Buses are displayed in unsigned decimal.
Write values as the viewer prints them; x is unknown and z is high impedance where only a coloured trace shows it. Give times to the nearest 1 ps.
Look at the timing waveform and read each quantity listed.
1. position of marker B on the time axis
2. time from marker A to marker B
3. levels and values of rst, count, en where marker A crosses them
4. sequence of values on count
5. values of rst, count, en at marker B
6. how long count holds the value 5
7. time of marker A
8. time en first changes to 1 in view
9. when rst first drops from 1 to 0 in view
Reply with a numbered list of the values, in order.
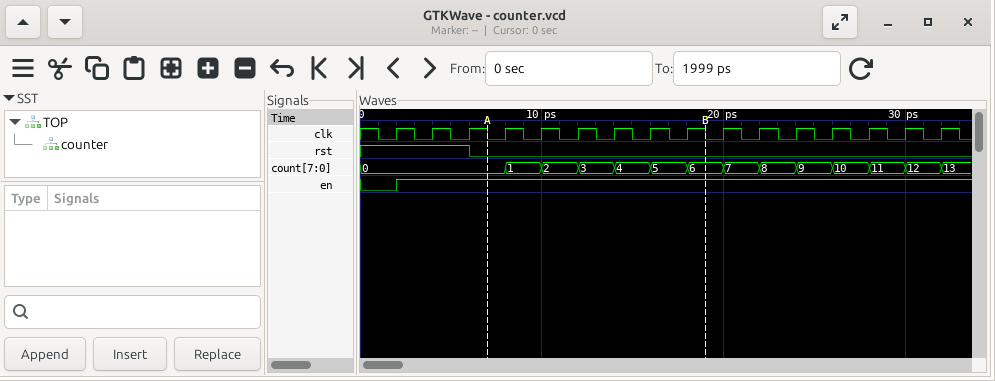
1. 19 ps
2. 12 ps
3. rst=0, count=0, en=1
4. 0, 1, 2, 3, 4, 5, 6, 7, 8, 9, 10, 11, 12, 13
5. rst=0, count=6, en=1
6. 2 ps
7. 7 ps
8. 2 ps
9. 6 ps
